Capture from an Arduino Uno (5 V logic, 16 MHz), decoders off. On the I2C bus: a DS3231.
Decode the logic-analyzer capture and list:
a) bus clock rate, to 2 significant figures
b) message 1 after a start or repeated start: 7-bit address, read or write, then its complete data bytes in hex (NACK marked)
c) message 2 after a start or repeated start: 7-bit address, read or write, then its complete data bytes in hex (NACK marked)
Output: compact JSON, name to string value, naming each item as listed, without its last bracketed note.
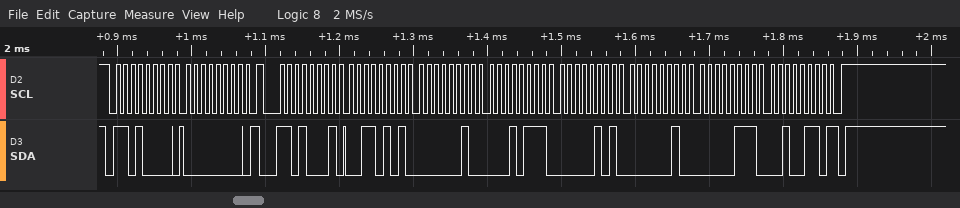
{"bus clock rate, to 2 significant figures": "100 kHz", "message 1 after a start or repeated start: 7-bit address, read or write, then its complete data bytes in hex": "0x68 write: 00", "message 2 after a start or repeated start: 7-bit address, read or write, then its complete data bytes in hex": "0x68 read: 35 02 17 05 02 07 26 NACK"}
